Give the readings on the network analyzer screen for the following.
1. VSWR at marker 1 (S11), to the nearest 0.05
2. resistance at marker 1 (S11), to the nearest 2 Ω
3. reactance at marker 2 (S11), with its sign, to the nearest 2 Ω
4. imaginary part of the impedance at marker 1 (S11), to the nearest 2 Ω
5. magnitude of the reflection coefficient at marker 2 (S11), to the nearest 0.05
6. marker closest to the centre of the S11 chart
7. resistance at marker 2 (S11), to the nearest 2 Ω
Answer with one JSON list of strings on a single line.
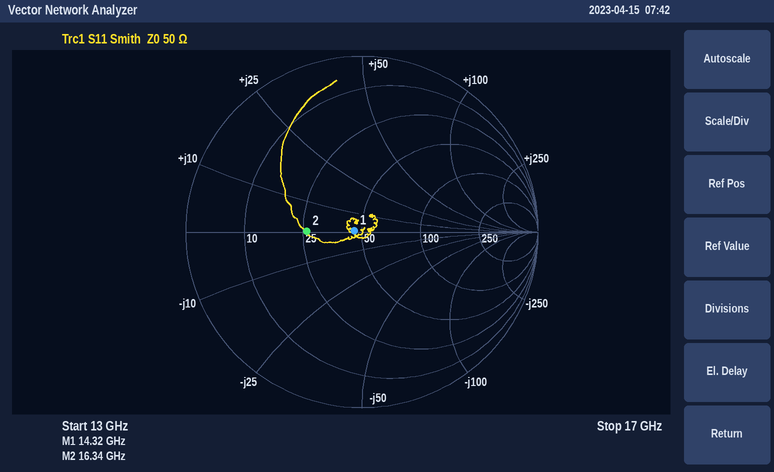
["1.10", "46 Ω", "0 Ω", "0 Ω", "0.30", "marker 1", "26 Ω"]
